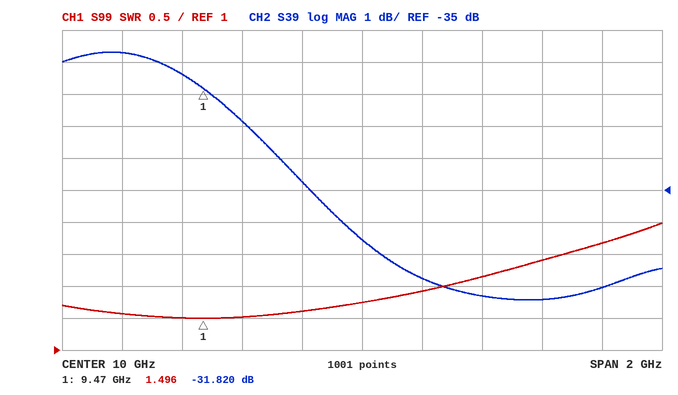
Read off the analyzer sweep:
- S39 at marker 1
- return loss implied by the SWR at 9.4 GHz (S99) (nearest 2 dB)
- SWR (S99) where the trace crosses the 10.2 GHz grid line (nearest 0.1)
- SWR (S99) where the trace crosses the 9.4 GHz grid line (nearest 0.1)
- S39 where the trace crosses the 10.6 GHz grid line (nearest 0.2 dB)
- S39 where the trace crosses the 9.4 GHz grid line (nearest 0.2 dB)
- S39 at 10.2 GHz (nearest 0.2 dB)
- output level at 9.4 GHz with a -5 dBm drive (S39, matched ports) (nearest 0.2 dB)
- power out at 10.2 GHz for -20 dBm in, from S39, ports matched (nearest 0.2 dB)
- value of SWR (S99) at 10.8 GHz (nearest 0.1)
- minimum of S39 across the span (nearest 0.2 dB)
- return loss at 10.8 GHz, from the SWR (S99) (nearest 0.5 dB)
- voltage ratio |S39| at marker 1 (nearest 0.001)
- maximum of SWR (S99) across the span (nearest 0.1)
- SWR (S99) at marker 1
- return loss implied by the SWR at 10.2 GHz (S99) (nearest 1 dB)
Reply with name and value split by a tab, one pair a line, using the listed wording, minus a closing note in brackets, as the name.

S39 at marker 1	-31.820 dB
return loss implied by the SWR at 9.4 GHz (S99)	14 dB
SWR (S99) where the trace crosses the 10.2 GHz grid line	1.9
SWR (S99) where the trace crosses the 9.4 GHz grid line	1.5
S39 where the trace crosses the 10.6 GHz grid line	-38.4 dB
S39 where the trace crosses the 9.4 GHz grid line	-31.4 dB
S39 at 10.2 GHz	-37.8 dB
output level at 9.4 GHz with a -5 dBm drive (S39, matched ports)	-36.4 dBm
power out at 10.2 GHz for -20 dBm in, from S39, ports matched	-57.8 dBm
value of SWR (S99) at 10.8 GHz	2.7
minimum of S39 across the span	-38.4 dB
return loss at 10.8 GHz, from the SWR (S99)	7.0 dB
voltage ratio |S39| at marker 1	0.026
maximum of SWR (S99) across the span	3.0
SWR (S99) at marker 1	1.496
return loss implied by the SWR at 10.2 GHz (S99)	10 dB
